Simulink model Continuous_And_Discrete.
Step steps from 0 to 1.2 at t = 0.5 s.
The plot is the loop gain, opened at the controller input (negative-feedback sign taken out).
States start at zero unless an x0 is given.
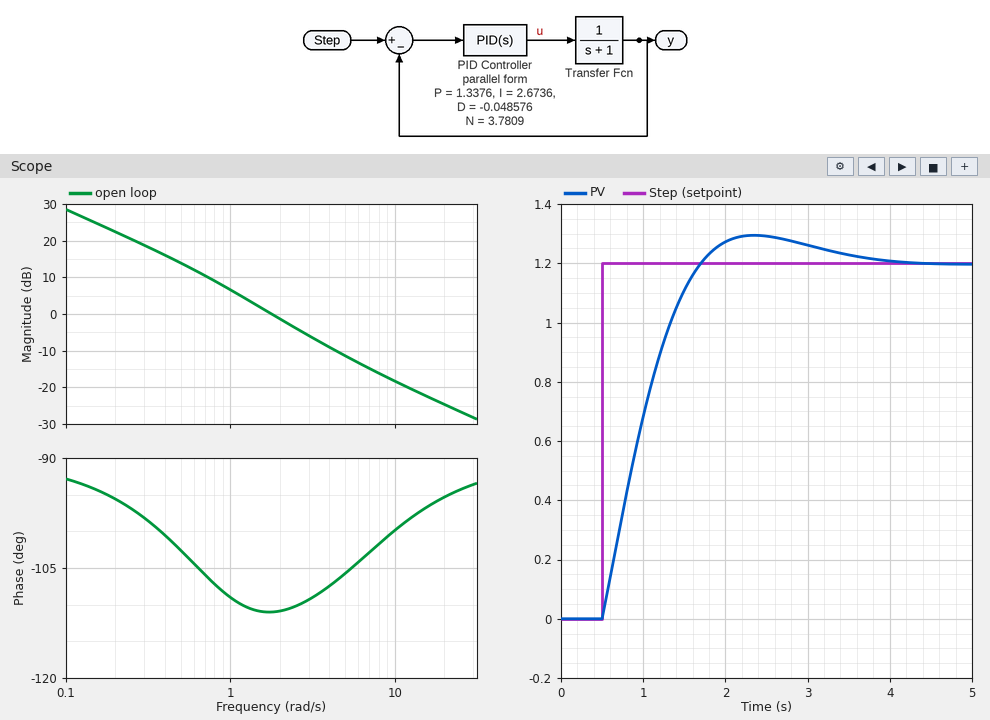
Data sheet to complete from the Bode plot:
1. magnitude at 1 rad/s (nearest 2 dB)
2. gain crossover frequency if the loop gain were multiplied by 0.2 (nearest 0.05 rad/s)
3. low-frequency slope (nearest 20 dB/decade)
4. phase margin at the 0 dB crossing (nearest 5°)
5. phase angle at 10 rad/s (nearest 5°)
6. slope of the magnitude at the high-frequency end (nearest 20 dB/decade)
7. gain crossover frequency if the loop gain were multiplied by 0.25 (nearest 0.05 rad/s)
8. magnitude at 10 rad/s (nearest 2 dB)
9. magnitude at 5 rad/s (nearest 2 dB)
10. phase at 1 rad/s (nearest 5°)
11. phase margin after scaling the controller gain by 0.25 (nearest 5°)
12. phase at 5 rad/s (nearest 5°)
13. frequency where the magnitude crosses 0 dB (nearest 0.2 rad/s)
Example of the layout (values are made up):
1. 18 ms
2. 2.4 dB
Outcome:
1. 6 dB
2. 0.50 rad/s
3. -20 dB/decade
4. 70°
5. -100°
6. -20 dB/decade
7. 0.60 rad/s
8. -18 dB
9. -12 dB
10. -110°
11. 75°
12. -105°
13. 1.8 rad/s
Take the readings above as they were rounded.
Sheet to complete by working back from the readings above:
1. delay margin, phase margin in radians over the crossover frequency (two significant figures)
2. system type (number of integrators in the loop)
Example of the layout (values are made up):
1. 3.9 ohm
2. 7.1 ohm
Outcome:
1. 0.68 s
2. 1
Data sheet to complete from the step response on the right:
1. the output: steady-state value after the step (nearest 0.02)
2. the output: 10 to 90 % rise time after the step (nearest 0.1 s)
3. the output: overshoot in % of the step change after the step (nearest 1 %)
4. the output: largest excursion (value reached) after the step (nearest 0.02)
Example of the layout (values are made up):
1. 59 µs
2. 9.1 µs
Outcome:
1. 1.20
2. 0.9 s
3. 8 %
4. 1.30
